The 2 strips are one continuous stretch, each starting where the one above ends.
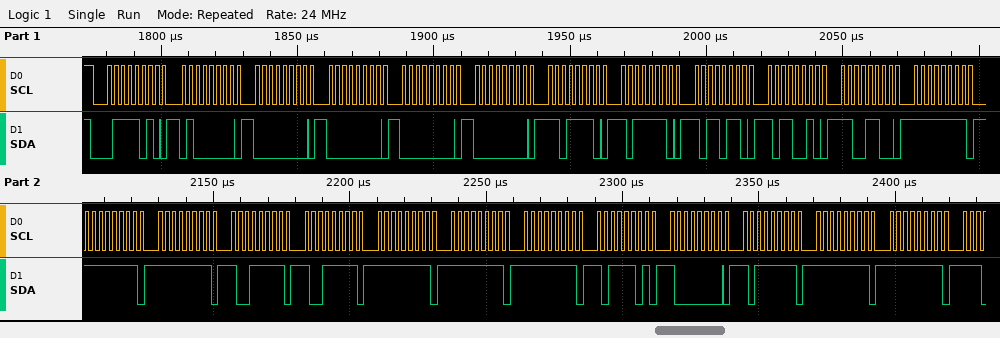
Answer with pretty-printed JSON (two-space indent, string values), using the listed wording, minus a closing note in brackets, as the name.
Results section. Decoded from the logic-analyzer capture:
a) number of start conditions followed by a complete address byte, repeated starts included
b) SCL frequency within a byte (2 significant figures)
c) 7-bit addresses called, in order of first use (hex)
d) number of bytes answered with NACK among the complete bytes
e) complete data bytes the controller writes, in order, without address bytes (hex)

{
  "number of start conditions followed by a complete address byte, repeated starts included": "1",
  "SCL frequency within a byte": "400 kHz",
  "7-bit addresses called, in order of first use": "0x3D",
  "number of bytes answered with NACK among the complete bytes": "0",
  "complete data bytes the controller writes, in order, without address bytes": "40 00 00 00 00 DE BE B6 B2 CC FF FF FF 9F 9F FF FF FF BD 80 BF FF FF"
}
